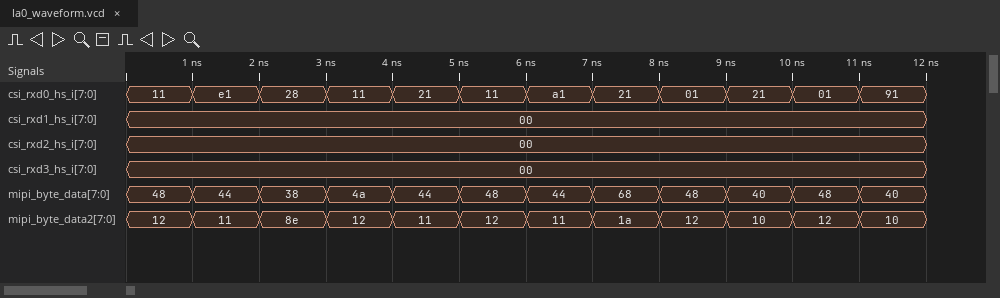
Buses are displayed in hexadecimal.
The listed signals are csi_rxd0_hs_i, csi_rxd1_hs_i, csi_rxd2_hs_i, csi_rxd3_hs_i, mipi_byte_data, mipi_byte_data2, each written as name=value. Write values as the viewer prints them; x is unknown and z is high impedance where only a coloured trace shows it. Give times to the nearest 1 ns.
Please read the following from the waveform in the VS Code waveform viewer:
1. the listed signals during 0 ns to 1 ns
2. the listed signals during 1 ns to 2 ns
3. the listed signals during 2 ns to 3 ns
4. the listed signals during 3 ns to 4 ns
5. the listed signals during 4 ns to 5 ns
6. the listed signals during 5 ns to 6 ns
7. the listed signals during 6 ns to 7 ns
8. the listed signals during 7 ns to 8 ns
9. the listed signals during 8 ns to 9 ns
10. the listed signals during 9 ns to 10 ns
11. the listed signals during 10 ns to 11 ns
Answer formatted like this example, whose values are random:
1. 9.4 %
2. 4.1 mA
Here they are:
1. csi_rxd0_hs_i=11, csi_rxd1_hs_i=00, csi_rxd2_hs_i=00, csi_rxd3_hs_i=00, mipi_byte_data=48, mipi_byte_data2=12
2. csi_rxd0_hs_i=e1, csi_rxd1_hs_i=00, csi_rxd2_hs_i=00, csi_rxd3_hs_i=00, mipi_byte_data=44, mipi_byte_data2=11
3. csi_rxd0_hs_i=28, csi_rxd1_hs_i=00, csi_rxd2_hs_i=00, csi_rxd3_hs_i=00, mipi_byte_data=38, mipi_byte_data2=8e
4. csi_rxd0_hs_i=11, csi_rxd1_hs_i=00, csi_rxd2_hs_i=00, csi_rxd3_hs_i=00, mipi_byte_data=4a, mipi_byte_data2=12
5. csi_rxd0_hs_i=21, csi_rxd1_hs_i=00, csi_rxd2_hs_i=00, csi_rxd3_hs_i=00, mipi_byte_data=44, mipi_byte_data2=11
6. csi_rxd0_hs_i=11, csi_rxd1_hs_i=00, csi_rxd2_hs_i=00, csi_rxd3_hs_i=00, mipi_byte_data=48, mipi_byte_data2=12
7. csi_rxd0_hs_i=a1, csi_rxd1_hs_i=00, csi_rxd2_hs_i=00, csi_rxd3_hs_i=00, mipi_byte_data=44, mipi_byte_data2=11
8. csi_rxd0_hs_i=21, csi_rxd1_hs_i=00, csi_rxd2_hs_i=00, csi_rxd3_hs_i=00, mipi_byte_data=68, mipi_byte_data2=1a
9. csi_rxd0_hs_i=01, csi_rxd1_hs_i=00, csi_rxd2_hs_i=00, csi_rxd3_hs_i=00, mipi_byte_data=48, mipi_byte_data2=12
10. csi_rxd0_hs_i=21, csi_rxd1_hs_i=00, csi_rxd2_hs_i=00, csi_rxd3_hs_i=00, mipi_byte_data=40, mipi_byte_data2=10
11. csi_rxd0_hs_i=01, csi_rxd1_hs_i=00, csi_rxd2_hs_i=00, csi_rxd3_hs_i=00, mipi_byte_data=48, mipi_byte_data2=12
